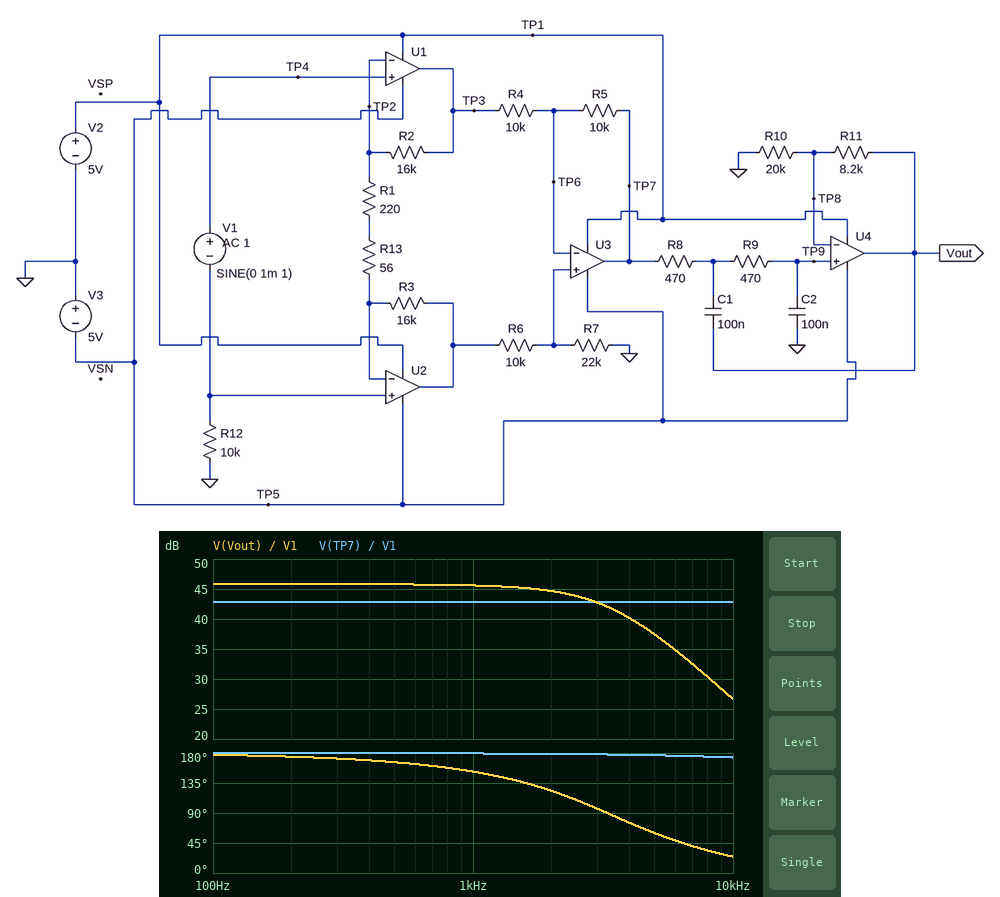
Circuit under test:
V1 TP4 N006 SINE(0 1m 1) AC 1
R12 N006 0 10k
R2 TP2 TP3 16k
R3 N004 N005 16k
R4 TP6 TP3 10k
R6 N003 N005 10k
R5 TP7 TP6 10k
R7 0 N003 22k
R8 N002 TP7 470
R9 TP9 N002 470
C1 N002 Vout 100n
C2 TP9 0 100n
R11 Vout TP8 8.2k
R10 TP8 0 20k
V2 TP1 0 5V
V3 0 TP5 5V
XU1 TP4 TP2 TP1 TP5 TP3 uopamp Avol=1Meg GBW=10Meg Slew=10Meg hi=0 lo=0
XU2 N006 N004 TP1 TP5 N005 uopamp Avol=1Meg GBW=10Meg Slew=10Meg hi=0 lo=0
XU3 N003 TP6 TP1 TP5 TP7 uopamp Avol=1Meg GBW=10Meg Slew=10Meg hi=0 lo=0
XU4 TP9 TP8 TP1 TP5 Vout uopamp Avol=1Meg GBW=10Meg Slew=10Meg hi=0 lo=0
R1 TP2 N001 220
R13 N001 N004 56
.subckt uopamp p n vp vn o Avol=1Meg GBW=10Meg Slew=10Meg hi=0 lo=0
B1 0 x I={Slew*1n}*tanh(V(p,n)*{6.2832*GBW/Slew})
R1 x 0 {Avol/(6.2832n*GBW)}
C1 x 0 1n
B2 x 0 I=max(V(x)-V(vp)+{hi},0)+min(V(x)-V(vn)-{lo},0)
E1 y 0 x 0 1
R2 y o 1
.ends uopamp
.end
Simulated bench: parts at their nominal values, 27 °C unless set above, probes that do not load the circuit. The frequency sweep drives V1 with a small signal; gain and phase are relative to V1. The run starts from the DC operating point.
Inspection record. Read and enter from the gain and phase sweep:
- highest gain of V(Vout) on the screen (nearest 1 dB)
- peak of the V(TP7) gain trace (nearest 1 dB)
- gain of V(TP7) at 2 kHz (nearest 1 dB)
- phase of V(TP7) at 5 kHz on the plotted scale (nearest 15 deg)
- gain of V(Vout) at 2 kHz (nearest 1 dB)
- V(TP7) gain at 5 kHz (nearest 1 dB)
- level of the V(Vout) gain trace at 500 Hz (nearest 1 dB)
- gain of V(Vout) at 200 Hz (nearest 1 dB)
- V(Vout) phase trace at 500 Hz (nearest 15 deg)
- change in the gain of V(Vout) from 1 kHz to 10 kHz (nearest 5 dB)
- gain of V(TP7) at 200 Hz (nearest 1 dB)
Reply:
46 dB
43 dB
43 dB
180 deg
45 dB
43 dB
46 dB
46 dB
165 deg
-20 dB
43 dB
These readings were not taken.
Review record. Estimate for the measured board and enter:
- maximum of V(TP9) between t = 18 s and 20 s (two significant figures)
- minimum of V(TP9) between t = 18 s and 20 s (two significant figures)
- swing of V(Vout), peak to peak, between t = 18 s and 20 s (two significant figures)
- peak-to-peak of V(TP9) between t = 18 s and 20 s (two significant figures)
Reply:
140 mV
-140 mV
390 mV
280 mV
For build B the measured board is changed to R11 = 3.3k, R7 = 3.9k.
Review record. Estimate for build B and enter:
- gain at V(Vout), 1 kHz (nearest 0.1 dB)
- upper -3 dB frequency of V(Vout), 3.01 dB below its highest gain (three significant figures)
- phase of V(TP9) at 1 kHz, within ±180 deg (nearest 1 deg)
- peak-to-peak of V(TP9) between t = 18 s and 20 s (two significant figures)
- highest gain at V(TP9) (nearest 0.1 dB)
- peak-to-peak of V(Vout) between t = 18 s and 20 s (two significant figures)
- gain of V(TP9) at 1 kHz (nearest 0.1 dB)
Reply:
40.0 dB
2.46 kHz
149 deg
180 mV
39.2 dB
210 mV
38.7 dB
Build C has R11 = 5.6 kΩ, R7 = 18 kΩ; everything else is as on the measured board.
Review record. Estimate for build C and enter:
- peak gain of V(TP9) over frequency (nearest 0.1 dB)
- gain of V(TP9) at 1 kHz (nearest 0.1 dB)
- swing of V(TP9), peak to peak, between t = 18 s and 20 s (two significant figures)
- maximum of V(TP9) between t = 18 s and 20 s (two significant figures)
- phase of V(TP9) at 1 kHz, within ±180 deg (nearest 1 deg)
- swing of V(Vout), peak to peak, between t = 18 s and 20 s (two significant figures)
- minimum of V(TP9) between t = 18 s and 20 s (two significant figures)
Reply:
42.5 dB
42.1 dB
270 mV
130 mV
150 deg
340 mV
-130 mV
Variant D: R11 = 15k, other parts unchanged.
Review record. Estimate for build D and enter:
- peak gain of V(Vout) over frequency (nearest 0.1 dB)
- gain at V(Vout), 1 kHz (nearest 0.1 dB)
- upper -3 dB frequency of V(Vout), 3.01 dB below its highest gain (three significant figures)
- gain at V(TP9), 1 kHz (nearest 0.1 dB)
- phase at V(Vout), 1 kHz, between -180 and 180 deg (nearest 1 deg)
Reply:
47.9 dB
47.8 dB
3.70 kHz
43.0 dB
157 deg
